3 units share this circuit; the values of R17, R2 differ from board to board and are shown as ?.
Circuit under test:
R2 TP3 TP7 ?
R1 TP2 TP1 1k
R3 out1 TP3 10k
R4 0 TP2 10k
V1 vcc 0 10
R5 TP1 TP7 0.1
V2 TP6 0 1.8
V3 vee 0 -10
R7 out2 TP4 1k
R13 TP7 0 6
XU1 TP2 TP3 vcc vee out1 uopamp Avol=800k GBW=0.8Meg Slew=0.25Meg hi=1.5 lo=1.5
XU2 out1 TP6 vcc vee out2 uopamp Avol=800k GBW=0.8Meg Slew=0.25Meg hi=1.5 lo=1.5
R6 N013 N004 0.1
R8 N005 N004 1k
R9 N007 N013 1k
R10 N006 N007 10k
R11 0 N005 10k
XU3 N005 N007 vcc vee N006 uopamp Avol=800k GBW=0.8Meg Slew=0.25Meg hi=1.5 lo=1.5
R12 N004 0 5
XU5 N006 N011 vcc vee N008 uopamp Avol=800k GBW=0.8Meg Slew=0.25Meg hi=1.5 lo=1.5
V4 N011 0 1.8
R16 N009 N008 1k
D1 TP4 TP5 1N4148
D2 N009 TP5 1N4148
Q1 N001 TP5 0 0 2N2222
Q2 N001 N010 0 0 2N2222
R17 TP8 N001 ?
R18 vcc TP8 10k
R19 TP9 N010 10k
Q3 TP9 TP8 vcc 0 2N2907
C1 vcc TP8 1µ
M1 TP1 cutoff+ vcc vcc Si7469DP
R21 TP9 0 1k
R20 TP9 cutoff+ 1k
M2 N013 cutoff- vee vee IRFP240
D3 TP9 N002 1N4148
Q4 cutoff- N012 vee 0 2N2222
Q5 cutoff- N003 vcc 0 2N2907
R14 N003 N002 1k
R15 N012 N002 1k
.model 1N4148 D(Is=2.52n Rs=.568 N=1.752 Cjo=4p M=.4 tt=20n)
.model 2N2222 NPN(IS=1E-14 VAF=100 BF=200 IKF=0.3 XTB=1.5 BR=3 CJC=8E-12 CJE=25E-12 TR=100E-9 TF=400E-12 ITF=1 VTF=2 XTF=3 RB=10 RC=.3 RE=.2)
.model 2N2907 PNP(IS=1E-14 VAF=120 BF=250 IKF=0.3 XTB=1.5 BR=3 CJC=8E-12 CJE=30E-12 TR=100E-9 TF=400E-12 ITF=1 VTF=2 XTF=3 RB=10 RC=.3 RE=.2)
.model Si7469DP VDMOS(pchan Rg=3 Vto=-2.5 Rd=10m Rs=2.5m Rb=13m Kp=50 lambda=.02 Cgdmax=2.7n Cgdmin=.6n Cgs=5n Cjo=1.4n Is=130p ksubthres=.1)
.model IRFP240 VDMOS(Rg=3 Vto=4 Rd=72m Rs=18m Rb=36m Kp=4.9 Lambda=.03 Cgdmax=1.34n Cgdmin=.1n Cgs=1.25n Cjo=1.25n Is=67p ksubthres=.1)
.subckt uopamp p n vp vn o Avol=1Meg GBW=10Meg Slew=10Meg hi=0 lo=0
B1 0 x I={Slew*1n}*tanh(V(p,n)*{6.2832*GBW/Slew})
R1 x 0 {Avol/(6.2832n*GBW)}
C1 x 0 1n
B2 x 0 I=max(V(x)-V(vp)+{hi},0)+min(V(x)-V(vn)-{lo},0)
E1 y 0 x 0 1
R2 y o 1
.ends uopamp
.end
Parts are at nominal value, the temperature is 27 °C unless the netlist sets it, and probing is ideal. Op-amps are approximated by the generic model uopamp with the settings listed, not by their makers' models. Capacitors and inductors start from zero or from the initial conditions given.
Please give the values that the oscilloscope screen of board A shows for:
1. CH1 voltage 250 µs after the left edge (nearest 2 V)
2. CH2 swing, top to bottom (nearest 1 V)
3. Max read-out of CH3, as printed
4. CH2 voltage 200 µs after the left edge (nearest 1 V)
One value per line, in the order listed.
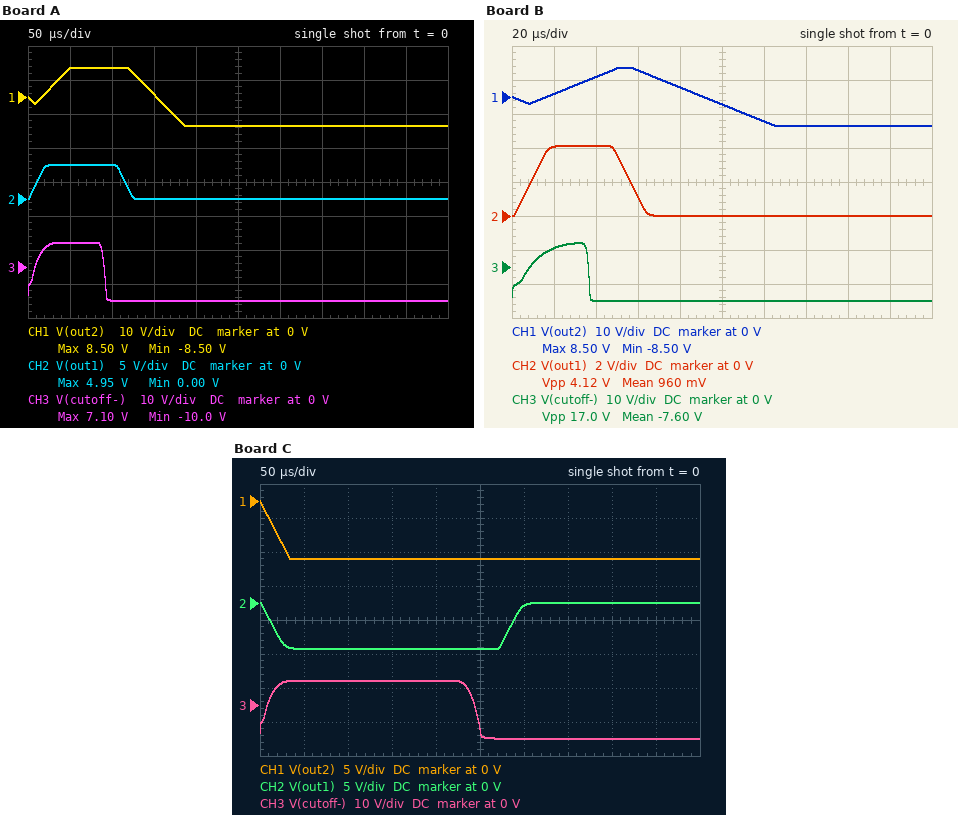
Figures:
-8 V
5 V
7.10 V
0 V
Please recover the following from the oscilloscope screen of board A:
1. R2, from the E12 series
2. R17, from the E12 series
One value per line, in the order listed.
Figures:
1.8 kΩ
1.2 kΩ
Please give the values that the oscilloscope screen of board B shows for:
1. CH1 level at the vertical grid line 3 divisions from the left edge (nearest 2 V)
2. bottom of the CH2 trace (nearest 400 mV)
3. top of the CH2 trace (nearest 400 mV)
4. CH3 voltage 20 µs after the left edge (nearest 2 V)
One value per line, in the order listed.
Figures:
8 V
0 V
4.0 V
6 V
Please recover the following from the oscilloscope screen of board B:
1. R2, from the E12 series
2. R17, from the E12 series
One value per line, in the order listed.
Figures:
1.5 kΩ
330 Ω
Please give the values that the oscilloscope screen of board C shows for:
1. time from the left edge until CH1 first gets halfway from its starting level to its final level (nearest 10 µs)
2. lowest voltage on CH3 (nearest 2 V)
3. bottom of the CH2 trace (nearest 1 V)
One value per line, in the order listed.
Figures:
20 µs
-10 V
-7 V
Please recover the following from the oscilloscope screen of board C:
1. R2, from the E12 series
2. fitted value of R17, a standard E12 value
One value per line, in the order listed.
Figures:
470 Ω
3.3 kΩ
